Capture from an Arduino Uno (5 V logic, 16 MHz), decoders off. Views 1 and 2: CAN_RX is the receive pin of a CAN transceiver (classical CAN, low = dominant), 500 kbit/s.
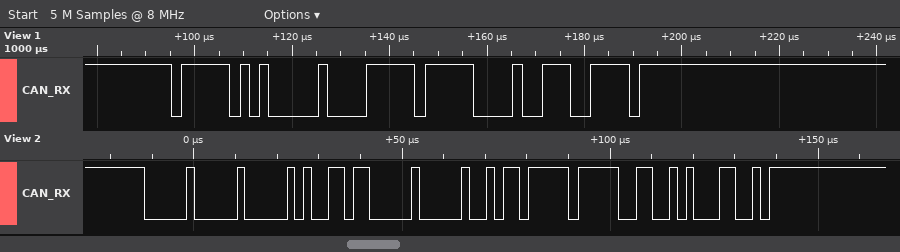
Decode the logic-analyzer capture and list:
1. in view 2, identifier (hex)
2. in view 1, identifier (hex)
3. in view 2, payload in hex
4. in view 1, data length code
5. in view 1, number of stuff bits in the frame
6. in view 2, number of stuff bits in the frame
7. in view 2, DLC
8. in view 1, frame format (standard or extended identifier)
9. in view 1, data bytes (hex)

0x000
0x7E8
D8 00 5B FF
1
4
7
4
standard
FF
